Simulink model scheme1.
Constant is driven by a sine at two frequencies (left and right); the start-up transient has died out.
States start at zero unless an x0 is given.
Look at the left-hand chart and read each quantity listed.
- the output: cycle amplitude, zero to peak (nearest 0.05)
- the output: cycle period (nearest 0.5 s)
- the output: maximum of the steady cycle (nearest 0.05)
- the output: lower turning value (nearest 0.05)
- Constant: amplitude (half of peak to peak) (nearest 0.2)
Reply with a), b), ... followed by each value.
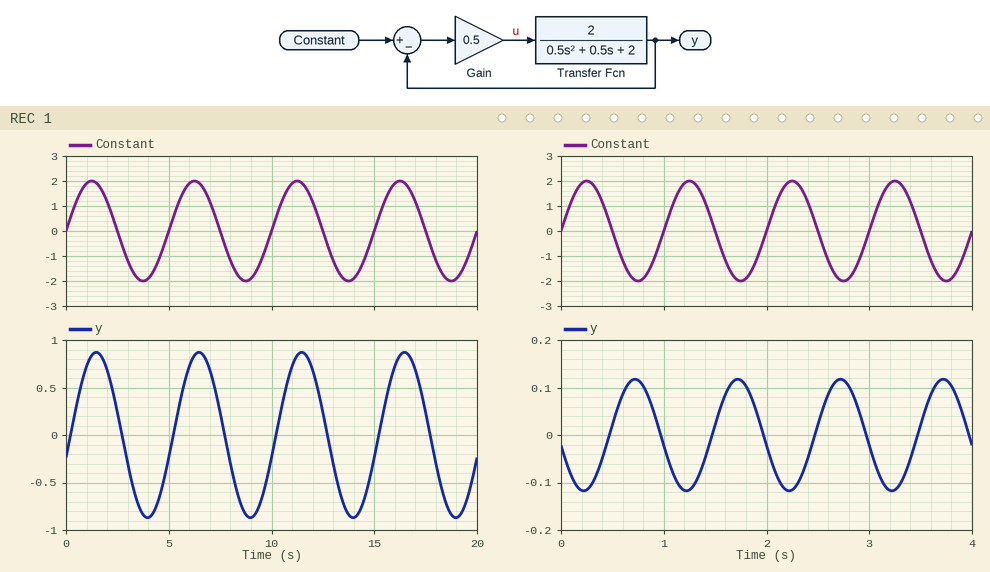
a) 0.85
b) 5.0 s
c) 0.85
d) -0.85
e) 2.0
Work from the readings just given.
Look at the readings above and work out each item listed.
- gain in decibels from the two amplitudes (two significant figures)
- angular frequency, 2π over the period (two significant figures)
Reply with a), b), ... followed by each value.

a) -7.4 dB
b) 1.3 rad/s
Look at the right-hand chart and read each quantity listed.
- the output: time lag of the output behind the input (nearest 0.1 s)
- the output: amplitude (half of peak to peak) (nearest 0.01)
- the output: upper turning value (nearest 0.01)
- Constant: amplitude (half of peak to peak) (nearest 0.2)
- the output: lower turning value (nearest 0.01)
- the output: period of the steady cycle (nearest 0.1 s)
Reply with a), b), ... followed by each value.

a) 0.5 s
b) 0.12
c) 0.12
d) 2.0
e) -0.12
f) 1.0 s
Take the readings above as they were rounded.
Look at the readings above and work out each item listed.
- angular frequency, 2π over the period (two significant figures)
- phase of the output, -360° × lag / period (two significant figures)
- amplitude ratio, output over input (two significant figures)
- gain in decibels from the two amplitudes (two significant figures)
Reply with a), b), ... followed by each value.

a) 6.3 rad/s
b) -180°
c) 0.060
d) -24 dB
